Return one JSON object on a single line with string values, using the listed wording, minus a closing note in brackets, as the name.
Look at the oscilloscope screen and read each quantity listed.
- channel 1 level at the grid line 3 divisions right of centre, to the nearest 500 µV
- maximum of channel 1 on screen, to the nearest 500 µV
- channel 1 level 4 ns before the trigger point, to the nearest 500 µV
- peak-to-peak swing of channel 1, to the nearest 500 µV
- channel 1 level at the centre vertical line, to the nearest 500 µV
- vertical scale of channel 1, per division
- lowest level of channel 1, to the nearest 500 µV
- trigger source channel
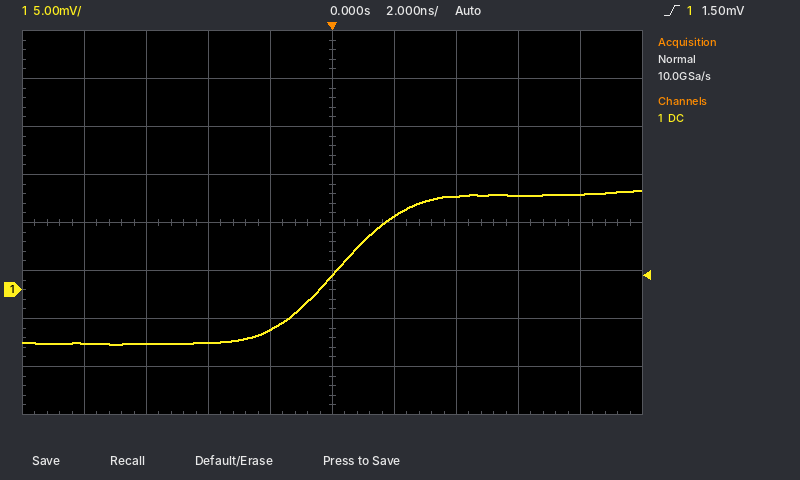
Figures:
{"channel 1 level at the grid line 3 divisions right of centre, to the nearest 500 µV": "10.0 mV", "maximum of channel 1 on screen, to the nearest 500 µV": "10.5 mV", "channel 1 level 4 ns before the trigger point, to the nearest 500 µV": "-5.5 mV", "peak-to-peak swing of channel 1, to the nearest 500 µV": "16.0 mV", "channel 1 level at the centre vertical line, to the nearest 500 µV": "1.5 mV", "vertical scale of channel 1, per division": "5 mV", "lowest level of channel 1, to the nearest 500 µV": "-5.5 mV", "trigger source channel": "channel 1"}
